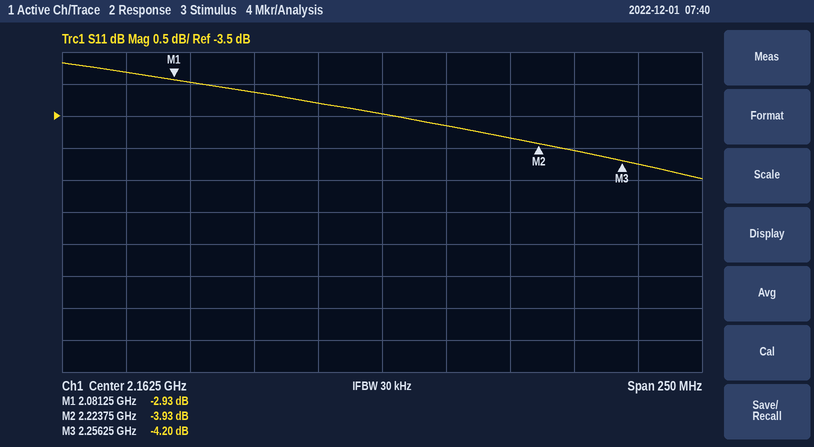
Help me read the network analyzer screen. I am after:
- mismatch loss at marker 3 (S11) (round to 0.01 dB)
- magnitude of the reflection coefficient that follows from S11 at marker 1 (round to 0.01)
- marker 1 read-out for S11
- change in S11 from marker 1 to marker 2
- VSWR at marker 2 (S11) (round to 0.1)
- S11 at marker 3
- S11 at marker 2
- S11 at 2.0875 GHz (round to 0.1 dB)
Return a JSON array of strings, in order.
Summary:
["2.08 dB", "0.71", "-2.93 dB", "-1.00 dB", "4.5", "-4.20 dB", "-3.93 dB", "-3.0 dB"]
